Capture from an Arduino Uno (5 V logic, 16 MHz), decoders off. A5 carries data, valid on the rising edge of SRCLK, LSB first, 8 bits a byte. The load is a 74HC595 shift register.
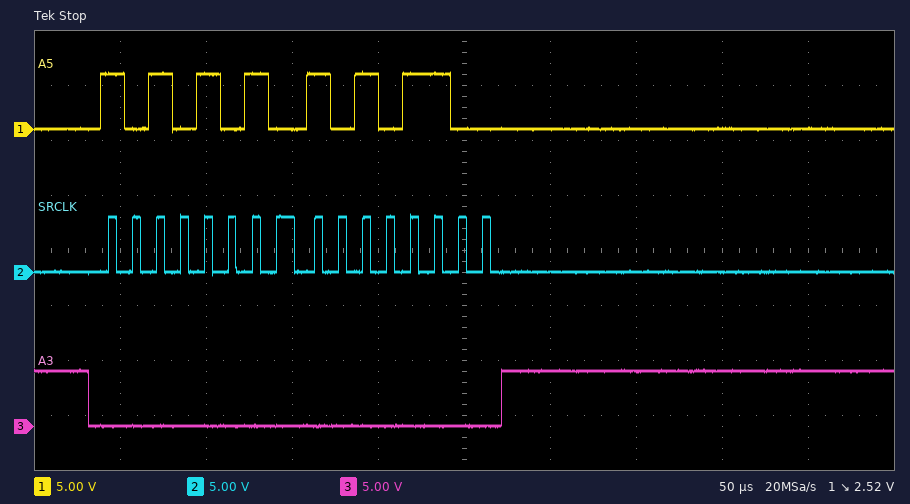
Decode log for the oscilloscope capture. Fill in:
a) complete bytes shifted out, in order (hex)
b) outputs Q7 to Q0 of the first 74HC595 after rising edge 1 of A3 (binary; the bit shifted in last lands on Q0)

55 35
10101100
